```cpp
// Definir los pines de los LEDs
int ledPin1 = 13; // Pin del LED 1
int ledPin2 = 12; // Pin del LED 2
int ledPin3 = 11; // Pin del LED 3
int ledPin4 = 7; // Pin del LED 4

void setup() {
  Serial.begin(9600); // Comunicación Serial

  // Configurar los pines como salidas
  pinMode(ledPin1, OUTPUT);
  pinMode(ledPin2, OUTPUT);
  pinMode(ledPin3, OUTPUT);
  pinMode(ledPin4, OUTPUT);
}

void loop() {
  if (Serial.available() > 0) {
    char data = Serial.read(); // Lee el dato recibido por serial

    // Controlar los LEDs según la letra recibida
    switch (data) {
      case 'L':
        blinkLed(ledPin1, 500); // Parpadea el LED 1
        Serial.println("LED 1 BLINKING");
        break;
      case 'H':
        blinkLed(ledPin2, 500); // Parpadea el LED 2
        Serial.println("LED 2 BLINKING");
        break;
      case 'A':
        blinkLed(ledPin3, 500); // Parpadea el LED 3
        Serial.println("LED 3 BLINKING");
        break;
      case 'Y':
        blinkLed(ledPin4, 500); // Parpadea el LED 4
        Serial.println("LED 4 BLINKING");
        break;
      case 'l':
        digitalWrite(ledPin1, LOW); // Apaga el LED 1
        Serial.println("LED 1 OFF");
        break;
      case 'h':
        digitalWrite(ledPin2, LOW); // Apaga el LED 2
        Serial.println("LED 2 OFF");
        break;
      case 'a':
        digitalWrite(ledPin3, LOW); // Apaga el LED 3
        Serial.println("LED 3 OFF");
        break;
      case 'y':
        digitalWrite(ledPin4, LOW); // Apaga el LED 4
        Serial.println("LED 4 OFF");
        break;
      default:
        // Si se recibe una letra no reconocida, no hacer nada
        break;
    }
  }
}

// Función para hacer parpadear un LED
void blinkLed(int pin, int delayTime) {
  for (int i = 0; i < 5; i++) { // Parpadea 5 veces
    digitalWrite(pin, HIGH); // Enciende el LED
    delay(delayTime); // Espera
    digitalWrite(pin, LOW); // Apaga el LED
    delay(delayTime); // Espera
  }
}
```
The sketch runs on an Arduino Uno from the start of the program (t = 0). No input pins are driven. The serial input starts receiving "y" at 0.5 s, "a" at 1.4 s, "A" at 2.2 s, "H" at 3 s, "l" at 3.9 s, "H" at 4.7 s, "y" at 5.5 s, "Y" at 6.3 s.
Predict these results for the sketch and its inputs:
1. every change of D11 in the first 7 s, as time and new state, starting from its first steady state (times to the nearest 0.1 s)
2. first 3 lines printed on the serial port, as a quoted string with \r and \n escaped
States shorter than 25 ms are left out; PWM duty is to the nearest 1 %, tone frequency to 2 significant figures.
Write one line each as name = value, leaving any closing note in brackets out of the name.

every change of D11 in the first 7 s, as time and new state, starting from its first steady state = 0 s low; 2.2 s high; 2.7 s low; 3.2 s high; 3.7 s low; 4.2 s high; 4.7 s low; 5.2 s high; 5.7 s low; 6.2 s high; 6.7 s low
first 3 lines printed on the serial port, as a quoted string with \r and \n escaped = "LED 4 OFF\r\nLED 3 OFF\r\nLED 3 BLINKING\r\n"
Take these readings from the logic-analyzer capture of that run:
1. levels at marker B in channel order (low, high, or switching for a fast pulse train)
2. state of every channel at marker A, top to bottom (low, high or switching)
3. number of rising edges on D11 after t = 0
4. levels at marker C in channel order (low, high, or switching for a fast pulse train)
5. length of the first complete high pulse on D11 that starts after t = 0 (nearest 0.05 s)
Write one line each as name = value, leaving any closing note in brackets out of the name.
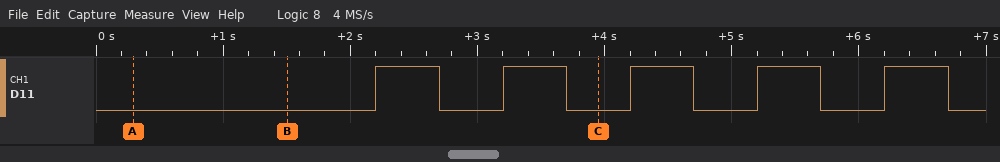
levels at marker B in channel order = D11 low
state of every channel at marker A, top to bottom = D11 low
number of rising edges on D11 after t = 0 = 5
levels at marker C in channel order = D11 low
length of the first complete high pulse on D11 that starts after t = 0 = 0.50 s
